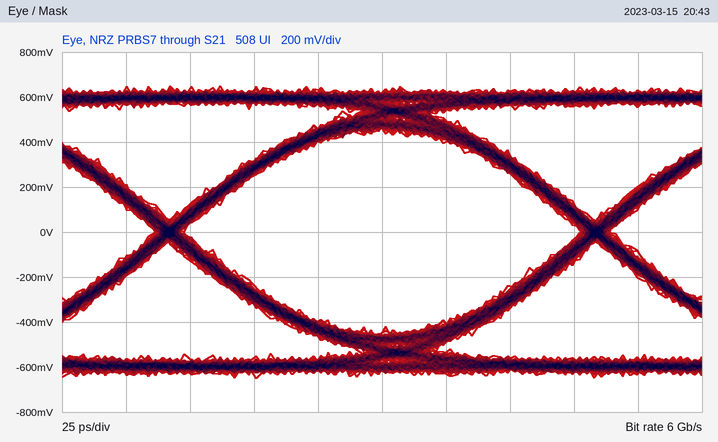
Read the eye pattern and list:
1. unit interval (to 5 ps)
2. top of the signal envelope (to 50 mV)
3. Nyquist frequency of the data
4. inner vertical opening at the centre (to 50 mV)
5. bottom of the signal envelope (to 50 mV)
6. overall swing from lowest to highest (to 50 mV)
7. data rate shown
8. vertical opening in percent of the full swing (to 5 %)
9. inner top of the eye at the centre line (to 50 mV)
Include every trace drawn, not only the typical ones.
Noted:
165 ps
650 mV
3 GHz
900 mV
-650 mV
1.30 V
6 Gb/s
70 %
450 mV
